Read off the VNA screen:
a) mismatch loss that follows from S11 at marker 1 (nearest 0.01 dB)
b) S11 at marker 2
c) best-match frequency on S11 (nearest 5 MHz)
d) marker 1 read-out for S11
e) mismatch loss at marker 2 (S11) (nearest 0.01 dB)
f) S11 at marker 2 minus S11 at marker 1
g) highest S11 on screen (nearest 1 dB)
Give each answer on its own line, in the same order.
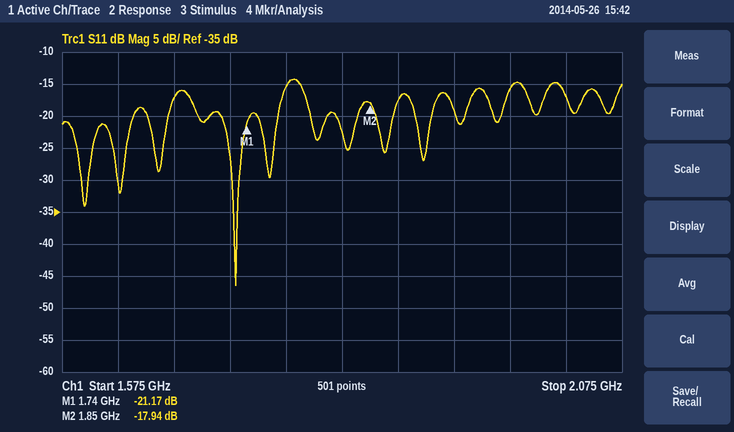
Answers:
0.03 dB
-17.94 dB
1.730 GHz
-21.17 dB
0.07 dB
3.23 dB
-14 dB
